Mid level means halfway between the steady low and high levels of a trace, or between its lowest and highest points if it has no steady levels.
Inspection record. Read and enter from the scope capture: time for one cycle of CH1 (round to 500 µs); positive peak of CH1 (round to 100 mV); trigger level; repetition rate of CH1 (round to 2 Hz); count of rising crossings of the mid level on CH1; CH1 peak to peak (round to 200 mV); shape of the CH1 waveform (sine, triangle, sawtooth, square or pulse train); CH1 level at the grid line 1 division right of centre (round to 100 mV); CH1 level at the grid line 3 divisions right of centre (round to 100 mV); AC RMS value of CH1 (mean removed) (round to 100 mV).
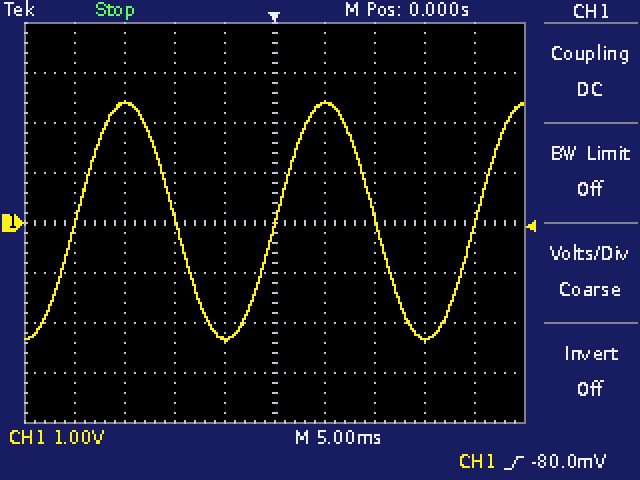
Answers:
20.0 ms
2.4 V
-80.0 mV
50 Hz
3
4.8 V
sine
2.4 V
-2.3 V
1.7 V
